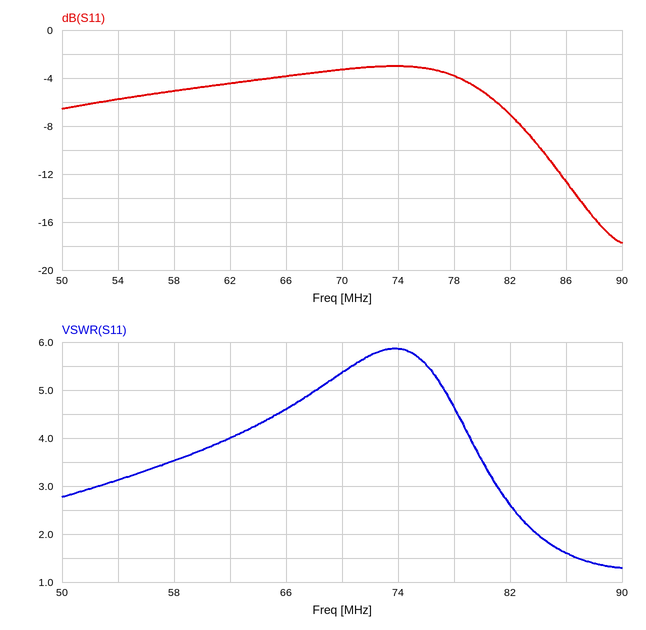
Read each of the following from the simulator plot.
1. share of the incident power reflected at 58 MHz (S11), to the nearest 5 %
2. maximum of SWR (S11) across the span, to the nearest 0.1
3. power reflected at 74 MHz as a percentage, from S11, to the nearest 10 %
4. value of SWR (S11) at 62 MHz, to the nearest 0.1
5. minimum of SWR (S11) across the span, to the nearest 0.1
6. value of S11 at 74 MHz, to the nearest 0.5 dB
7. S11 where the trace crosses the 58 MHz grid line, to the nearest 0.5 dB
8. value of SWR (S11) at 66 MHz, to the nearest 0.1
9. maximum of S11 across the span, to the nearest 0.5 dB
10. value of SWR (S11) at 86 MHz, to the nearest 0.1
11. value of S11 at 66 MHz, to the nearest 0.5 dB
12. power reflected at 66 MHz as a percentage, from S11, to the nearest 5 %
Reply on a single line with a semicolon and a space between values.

30 %; 5.9; 50 %; 4.0; 1.3; -3.0 dB; -5.0 dB; 4.6; -3.0 dB; 1.6; -4.0 dB; 40 %
